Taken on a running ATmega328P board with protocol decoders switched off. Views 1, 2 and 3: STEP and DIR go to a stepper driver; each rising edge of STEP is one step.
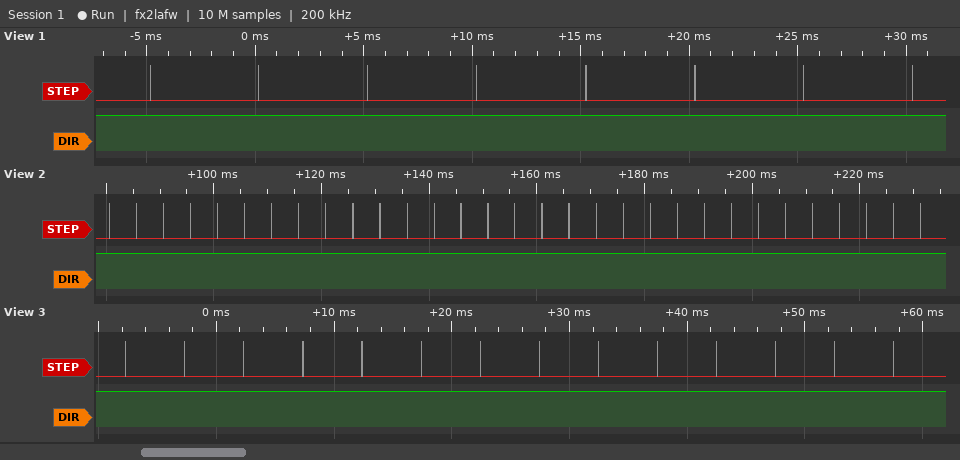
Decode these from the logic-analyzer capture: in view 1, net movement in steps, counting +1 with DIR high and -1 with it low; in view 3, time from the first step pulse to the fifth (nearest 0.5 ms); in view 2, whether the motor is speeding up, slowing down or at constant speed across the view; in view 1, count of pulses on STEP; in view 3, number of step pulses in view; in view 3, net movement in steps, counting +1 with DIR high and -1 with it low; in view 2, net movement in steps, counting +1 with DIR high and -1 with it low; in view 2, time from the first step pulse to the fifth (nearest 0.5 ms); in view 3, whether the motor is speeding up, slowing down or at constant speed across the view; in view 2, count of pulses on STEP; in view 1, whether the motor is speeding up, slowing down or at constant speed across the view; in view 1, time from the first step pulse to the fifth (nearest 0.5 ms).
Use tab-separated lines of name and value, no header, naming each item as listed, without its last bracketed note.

in view 1, net movement in steps, counting +1 with DIR high and -1 with it low	+8
in view 3, time from the first step pulse to the fifth	20.0 ms
in view 2, whether the motor is speeding up, slowing down or at constant speed across the view	constant speed
in view 1, count of pulses on STEP	8
in view 3, number of step pulses in view	14
in view 3, net movement in steps, counting +1 with DIR high and -1 with it low	+14
in view 2, net movement in steps, counting +1 with DIR high and -1 with it low	+31
in view 2, time from the first step pulse to the fifth	20.0 ms
in view 3, whether the motor is speeding up, slowing down or at constant speed across the view	constant speed
in view 2, count of pulses on STEP	31
in view 1, whether the motor is speeding up, slowing down or at constant speed across the view	constant speed
in view 1, time from the first step pulse to the fifth	20.0 ms
